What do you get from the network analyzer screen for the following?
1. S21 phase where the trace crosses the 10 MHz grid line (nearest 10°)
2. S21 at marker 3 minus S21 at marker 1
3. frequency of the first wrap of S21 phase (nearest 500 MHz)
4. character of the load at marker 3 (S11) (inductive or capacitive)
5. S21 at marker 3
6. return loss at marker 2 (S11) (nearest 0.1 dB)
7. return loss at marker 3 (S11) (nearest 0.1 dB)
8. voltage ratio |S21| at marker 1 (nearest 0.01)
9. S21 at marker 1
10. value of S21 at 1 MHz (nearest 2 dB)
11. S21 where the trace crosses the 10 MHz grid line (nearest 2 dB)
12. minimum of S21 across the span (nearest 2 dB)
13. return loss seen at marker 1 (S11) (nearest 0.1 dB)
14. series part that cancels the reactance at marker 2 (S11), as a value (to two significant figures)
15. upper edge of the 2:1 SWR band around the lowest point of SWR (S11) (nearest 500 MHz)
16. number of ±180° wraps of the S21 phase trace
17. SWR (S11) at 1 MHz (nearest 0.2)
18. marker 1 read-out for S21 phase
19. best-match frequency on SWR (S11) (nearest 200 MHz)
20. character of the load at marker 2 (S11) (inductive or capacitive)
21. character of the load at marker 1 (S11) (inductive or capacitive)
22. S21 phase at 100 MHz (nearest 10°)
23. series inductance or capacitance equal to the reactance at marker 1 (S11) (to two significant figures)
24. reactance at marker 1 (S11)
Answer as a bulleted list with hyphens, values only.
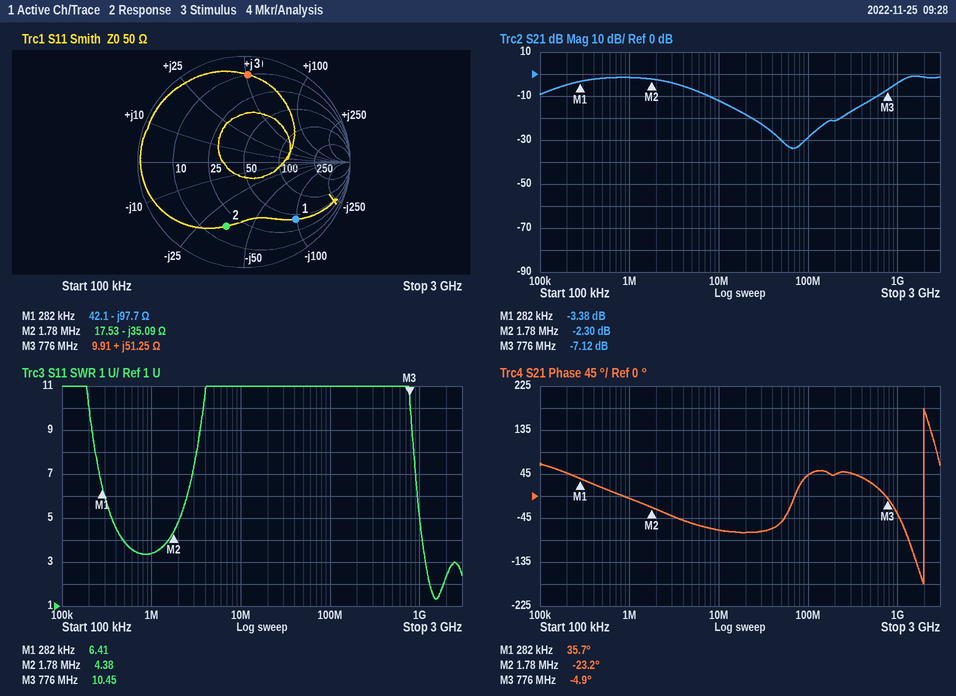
- -70°
- -3.74 dB
- 2.0 GHz
- inductive
- -7.12 dB
- 4.0 dB
- 1.7 dB
- 0.68
- -3.38 dB
- -2 dB
- -12 dB
- -34 dB
- 2.7 dB
- 3.1 µH
- 2.0 GHz
- 1
- 3.4
- 35.7°
- 1.6 GHz
- capacitive
- capacitive
- 40°
- 5.8 nF
- -97.7 Ω
